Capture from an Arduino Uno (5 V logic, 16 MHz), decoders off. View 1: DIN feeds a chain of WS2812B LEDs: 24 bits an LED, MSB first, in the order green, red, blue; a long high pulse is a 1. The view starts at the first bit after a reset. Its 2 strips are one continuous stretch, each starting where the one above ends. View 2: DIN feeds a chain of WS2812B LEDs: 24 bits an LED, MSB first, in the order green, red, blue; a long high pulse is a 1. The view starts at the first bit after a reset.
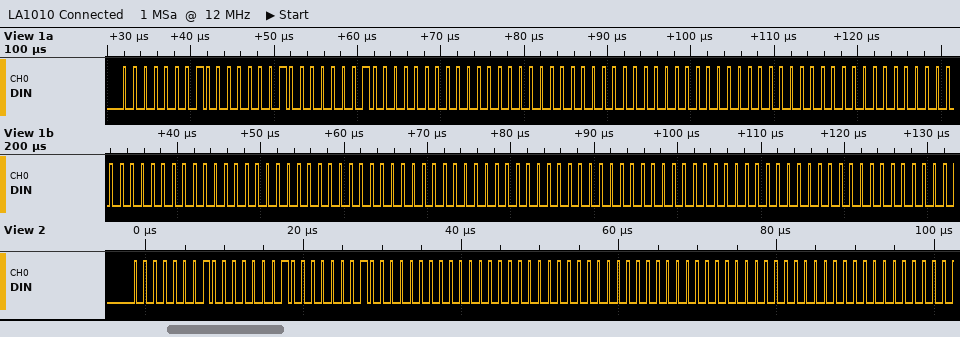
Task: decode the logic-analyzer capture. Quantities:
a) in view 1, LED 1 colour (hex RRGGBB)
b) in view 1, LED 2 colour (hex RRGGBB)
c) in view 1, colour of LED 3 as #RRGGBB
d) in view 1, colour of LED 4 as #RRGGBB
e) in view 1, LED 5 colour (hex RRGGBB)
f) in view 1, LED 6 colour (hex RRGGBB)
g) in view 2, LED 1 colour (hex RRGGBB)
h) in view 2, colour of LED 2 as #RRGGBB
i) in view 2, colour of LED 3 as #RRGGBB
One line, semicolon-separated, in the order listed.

#010101; #000000; #000000; #000000; #000000; #000000; #010101; #000000; #000000
